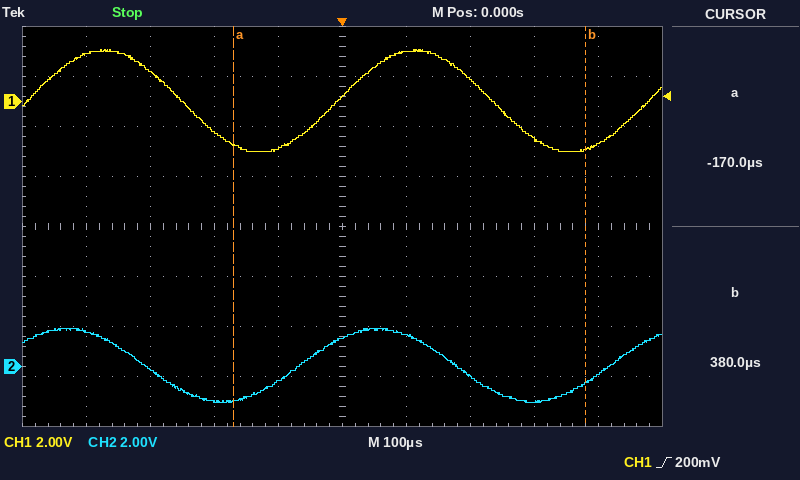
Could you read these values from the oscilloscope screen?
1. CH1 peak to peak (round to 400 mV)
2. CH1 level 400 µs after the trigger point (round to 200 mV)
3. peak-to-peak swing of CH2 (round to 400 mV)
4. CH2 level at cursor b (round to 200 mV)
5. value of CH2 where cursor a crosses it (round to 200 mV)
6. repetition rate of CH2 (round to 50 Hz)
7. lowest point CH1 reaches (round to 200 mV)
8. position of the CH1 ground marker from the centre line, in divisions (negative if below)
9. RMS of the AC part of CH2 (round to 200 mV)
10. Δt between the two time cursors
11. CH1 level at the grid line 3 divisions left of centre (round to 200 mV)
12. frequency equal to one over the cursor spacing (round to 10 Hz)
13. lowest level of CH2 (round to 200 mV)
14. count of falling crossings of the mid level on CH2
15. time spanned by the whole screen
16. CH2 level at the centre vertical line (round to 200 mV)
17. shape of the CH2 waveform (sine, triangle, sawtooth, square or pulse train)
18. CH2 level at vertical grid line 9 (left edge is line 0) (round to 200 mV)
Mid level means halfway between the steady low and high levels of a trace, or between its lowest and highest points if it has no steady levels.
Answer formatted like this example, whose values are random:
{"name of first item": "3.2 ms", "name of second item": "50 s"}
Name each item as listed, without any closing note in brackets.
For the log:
{"CH1 peak to peak": "4.0 V", "CH1 level 400 µs after the trigger point": "-1.6 V", "peak-to-peak swing of CH2": "2.8 V", "CH2 level at cursor b": "-600 mV", "value of CH2 where cursor a crosses it": "-1.4 V", "repetition rate of CH2": "2.05 kHz", "lowest point CH1 reaches": "-2.0 V", "position of the CH1 ground marker from the centre line, in divisions": "+2.5 div", "RMS of the AC part of CH2": "1.0 V", "Δt between the two time cursors": "550 µs", "CH1 level at the grid line 3 divisions left of centre": "1.2 V", "frequency equal to one over the cursor spacing": "1.82 kHz", "lowest level of CH2": "-1.4 V", "count of falling crossings of the mid level on CH2": "2", "time spanned by the whole screen": "1 ms", "CH2 level at the centre vertical line": "1.2 V", "shape of the CH2 waveform": "sine", "CH2 level at vertical grid line 9 (left edge is line 0)": "-400 mV"}
